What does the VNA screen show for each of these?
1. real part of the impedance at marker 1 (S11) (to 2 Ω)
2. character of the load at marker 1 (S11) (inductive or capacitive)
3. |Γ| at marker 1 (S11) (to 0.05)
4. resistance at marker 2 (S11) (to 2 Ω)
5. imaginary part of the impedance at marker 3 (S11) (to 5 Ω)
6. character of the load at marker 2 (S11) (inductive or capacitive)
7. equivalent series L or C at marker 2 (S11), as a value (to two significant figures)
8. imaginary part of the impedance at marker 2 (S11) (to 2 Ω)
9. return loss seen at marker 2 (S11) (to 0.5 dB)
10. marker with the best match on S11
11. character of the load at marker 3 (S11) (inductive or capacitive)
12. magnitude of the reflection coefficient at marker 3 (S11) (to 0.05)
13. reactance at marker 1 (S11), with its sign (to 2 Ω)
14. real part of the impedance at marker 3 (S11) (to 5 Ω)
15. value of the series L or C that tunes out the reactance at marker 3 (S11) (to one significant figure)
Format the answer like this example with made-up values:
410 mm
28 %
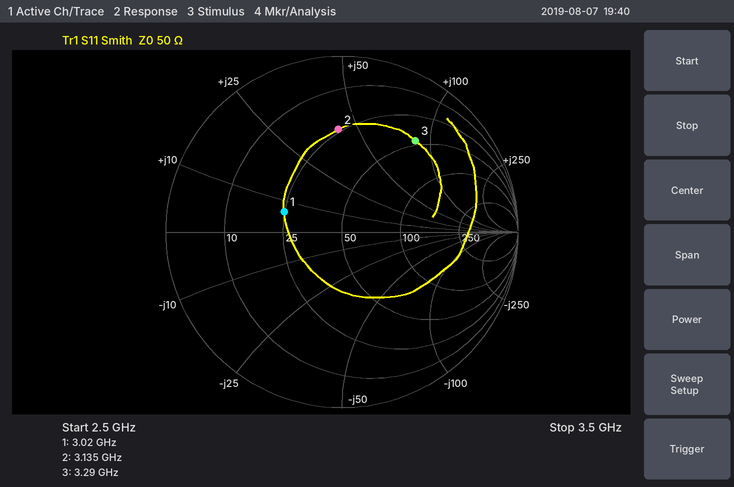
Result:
24 Ω
inductive
0.35
24 Ω
+85 Ω
inductive
2.1 nH
+42 Ω
4.5 dB
marker 1
inductive
0.65
+6 Ω
45 Ω
600 fF
